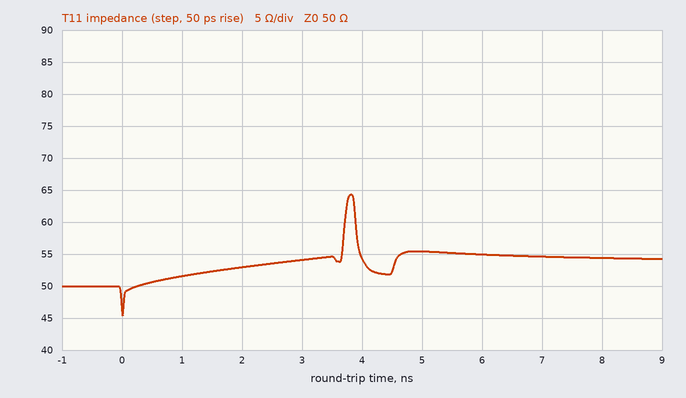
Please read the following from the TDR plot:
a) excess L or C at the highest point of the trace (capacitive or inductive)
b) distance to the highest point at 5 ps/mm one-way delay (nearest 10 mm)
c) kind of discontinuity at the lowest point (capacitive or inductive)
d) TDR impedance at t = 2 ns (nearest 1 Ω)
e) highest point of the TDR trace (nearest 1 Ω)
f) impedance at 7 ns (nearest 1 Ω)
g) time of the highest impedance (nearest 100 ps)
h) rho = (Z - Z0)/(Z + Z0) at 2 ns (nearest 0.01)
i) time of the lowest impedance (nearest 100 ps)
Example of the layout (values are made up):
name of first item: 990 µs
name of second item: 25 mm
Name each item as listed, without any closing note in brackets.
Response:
excess L or C at the highest point of the trace: inductive
distance to the highest point at 5 ps/mm one-way delay: 380 mm
kind of discontinuity at the lowest point: capacitive
TDR impedance at t = 2 ns: 53 Ω
highest point of the TDR trace: 64 Ω
impedance at 7 ns: 55 Ω
time of the highest impedance: 3.8 ns
rho = (Z - Z0)/(Z + Z0) at 2 ns: +0.03
time of the lowest impedance: 0.0 ns
